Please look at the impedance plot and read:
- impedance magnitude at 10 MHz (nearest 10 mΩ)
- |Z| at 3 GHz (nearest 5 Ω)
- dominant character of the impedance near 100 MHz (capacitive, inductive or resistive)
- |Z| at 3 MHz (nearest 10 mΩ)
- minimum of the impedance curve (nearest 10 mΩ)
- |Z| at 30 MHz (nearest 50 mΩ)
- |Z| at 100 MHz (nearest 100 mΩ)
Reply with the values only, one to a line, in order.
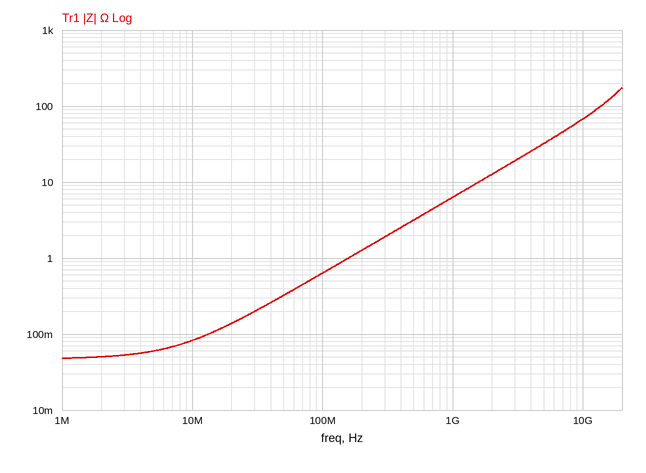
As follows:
80 mΩ
20 Ω
inductive
50 mΩ
50 mΩ
200 mΩ
600 mΩ
